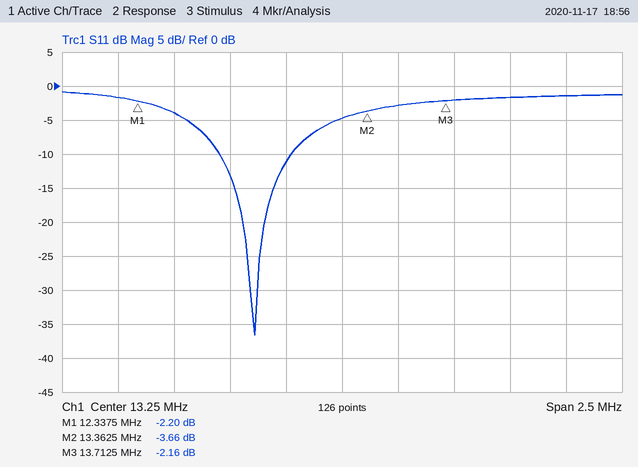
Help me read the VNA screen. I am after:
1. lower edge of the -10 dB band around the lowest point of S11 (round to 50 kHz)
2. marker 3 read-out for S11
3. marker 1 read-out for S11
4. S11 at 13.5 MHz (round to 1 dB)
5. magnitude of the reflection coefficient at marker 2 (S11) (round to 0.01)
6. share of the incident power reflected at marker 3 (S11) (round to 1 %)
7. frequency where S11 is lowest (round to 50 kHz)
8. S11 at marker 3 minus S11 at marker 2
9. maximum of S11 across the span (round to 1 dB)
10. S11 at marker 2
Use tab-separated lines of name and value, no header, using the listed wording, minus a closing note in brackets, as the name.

lower edge of the -10 dB band around the lowest point of S11	12.70 MHz
marker 3 read-out for S11	-2.16 dB
marker 1 read-out for S11	-2.20 dB
S11 at 13.5 MHz	-3 dB
magnitude of the reflection coefficient at marker 2 (S11)	0.66
share of the incident power reflected at marker 3 (S11)	61 %
frequency where S11 is lowest	12.85 MHz
S11 at marker 3 minus S11 at marker 2	1.50 dB
maximum of S11 across the span	-1 dB
S11 at marker 2	-3.66 dB
